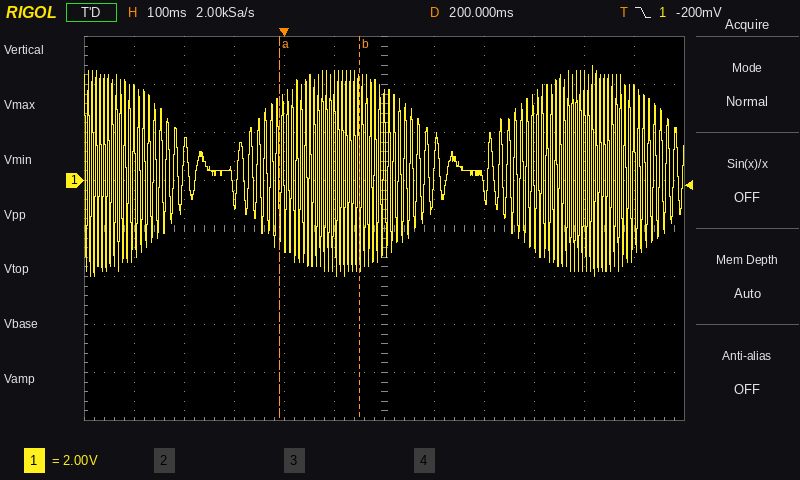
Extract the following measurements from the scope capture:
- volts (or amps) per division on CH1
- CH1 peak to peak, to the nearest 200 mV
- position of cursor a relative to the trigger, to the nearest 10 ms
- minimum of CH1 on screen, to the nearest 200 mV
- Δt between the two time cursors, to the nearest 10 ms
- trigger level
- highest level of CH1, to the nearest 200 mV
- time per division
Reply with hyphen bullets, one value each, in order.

- 2 V
- 8.8 V
- -10 ms
- -4.0 V
- 160 ms
- -200 mV
- 4.8 V
- 100 ms
